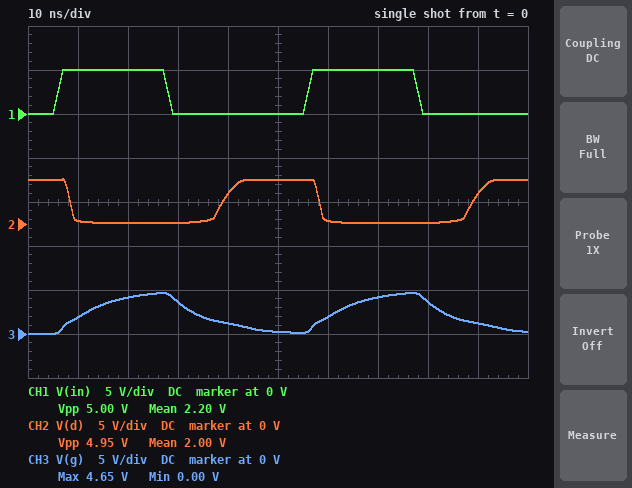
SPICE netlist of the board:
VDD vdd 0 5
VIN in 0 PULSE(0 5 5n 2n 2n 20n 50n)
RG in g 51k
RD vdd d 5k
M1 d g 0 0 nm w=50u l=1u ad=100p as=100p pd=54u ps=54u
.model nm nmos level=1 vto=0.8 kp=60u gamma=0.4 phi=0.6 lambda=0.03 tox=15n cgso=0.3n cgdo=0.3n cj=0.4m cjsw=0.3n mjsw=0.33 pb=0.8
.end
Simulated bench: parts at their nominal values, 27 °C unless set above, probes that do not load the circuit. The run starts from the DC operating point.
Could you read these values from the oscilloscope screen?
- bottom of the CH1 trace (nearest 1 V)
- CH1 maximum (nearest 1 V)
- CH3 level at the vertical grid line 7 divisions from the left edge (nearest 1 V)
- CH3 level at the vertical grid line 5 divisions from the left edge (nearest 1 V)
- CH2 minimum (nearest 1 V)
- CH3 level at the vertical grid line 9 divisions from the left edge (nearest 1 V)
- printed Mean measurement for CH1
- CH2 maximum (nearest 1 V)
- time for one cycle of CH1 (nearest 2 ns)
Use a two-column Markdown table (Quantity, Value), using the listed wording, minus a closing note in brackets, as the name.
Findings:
| Quantity | Value |
|---|---|
| bottom of the CH1 trace | 0 V |
| CH1 maximum | 5 V |
| CH3 level at the vertical grid line 7 divisions from the left edge | 4 V |
| CH3 level at the vertical grid line 5 divisions from the left edge | 0 V |
| CH2 minimum | 0 V |
| CH3 level at the vertical grid line 9 divisions from the left edge | 1 V |
| printed Mean measurement for CH1 | 2.20 V |
| CH2 maximum | 5 V |
| time for one cycle of CH1 | 50 ns |
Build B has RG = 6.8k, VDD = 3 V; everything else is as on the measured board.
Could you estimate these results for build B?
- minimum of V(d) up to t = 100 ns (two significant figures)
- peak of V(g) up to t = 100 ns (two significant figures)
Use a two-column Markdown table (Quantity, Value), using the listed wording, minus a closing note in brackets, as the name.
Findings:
| Quantity | Value |
|---|---|
| minimum of V(d) up to t = 100 ns | 44 mV |
| peak of V(g) up to t = 100 ns | 5.0 V |
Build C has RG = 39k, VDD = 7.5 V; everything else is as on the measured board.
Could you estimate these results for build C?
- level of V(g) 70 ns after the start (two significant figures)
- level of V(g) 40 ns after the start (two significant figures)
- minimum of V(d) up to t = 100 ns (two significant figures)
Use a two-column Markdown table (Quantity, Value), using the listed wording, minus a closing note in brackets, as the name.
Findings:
| Quantity | Value |
|---|---|
| level of V(g) 70 ns after the start | 4.5 V |
| level of V(g) 40 ns after the start | 920 mV |
| minimum of V(d) up to t = 100 ns | 120 mV |
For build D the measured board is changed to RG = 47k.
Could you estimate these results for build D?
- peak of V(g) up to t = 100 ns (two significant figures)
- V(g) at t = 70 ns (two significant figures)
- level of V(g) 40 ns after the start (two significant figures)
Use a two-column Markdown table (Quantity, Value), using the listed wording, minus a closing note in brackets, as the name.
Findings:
| Quantity | Value |
|---|---|
| peak of V(g) up to t = 100 ns | 4.7 V |
| V(g) at t = 70 ns | 4.3 V |
| level of V(g) 40 ns after the start | 1.1 V |
